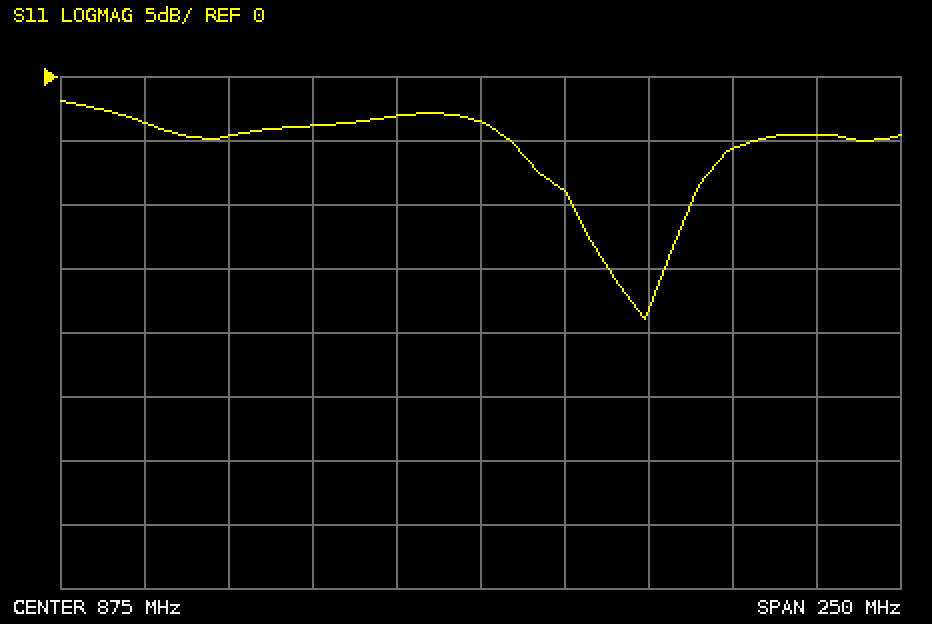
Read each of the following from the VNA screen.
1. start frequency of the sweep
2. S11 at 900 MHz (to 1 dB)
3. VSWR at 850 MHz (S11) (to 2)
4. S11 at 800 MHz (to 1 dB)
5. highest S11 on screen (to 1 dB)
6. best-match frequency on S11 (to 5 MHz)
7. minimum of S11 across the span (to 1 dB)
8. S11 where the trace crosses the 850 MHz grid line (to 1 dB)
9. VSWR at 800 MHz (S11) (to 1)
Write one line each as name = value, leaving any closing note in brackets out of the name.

start frequency of the sweep = 750 MHz
S11 at 900 MHz = -9 dB
VSWR at 850 MHz (S11) = 6
S11 at 800 MHz = -5 dB
highest S11 on screen = -2 dB
best-match frequency on S11 = 925 MHz
minimum of S11 across the span = -19 dB
S11 where the trace crosses the 850 MHz grid line = -3 dB
VSWR at 800 MHz (S11) = 4
